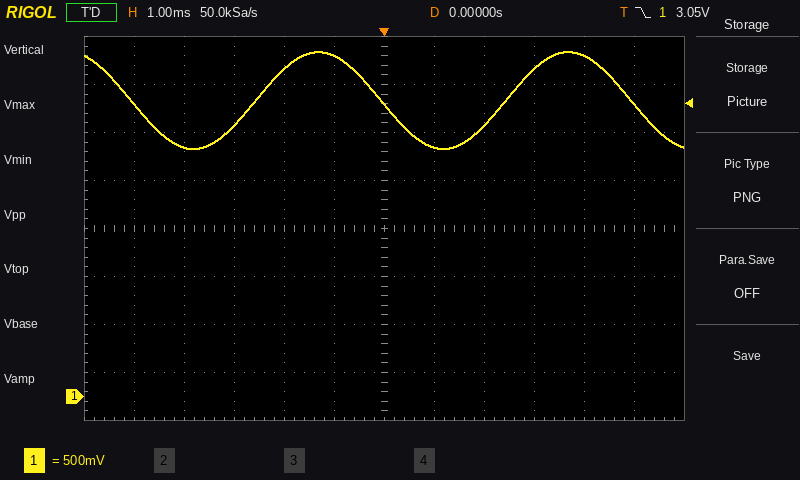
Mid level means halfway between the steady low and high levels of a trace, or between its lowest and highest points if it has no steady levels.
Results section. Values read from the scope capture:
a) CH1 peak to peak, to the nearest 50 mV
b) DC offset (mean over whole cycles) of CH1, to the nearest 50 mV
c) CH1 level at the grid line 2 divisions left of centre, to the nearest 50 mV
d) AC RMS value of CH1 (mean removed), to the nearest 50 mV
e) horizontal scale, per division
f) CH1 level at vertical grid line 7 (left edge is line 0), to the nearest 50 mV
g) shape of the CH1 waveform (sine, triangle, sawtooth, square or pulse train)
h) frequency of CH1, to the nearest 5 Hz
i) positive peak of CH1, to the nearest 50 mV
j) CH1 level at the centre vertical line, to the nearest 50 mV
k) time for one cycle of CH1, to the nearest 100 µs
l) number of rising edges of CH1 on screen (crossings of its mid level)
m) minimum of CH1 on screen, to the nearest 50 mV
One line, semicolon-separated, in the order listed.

1.00 V; 3.10 V; 3.40 V; 350 mV; 1 ms; 2.60 V; sine; 200 Hz; 3.60 V; 3.05 V; 5.0 ms; 2; 2.60 V
